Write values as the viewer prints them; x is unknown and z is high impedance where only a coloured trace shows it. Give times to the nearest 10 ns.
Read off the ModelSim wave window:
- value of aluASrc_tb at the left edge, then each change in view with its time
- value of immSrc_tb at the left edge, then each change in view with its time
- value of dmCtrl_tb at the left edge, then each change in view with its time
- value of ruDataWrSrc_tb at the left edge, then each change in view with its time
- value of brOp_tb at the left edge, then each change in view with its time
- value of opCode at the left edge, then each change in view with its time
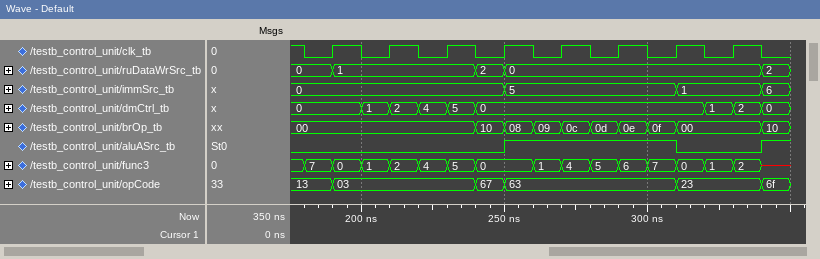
0, 1 at 250 ns, 0 at 310 ns, 1 at 340 ns
0, 5 at 250 ns, 1 at 310 ns, 6 at 340 ns
0, 1 at 200 ns, 2 at 210 ns, 4 at 220 ns, 5 at 230 ns, 0 at 240 ns, 1 at 320 ns, 2 at 330 ns, 0 at 340 ns
0, 1 at 190 ns, 2 at 240 ns, 0 at 250 ns, 2 at 340 ns
00, 10 at 240 ns, 08 at 250 ns, 09 at 260 ns, 0c at 270 ns, 0d at 280 ns, 0e at 290 ns, 0f at 300 ns, 00 at 310 ns, 10 at 340 ns
13, 03 at 190 ns, 67 at 240 ns, 63 at 250 ns, 23 at 310 ns, 6f at 340 ns
